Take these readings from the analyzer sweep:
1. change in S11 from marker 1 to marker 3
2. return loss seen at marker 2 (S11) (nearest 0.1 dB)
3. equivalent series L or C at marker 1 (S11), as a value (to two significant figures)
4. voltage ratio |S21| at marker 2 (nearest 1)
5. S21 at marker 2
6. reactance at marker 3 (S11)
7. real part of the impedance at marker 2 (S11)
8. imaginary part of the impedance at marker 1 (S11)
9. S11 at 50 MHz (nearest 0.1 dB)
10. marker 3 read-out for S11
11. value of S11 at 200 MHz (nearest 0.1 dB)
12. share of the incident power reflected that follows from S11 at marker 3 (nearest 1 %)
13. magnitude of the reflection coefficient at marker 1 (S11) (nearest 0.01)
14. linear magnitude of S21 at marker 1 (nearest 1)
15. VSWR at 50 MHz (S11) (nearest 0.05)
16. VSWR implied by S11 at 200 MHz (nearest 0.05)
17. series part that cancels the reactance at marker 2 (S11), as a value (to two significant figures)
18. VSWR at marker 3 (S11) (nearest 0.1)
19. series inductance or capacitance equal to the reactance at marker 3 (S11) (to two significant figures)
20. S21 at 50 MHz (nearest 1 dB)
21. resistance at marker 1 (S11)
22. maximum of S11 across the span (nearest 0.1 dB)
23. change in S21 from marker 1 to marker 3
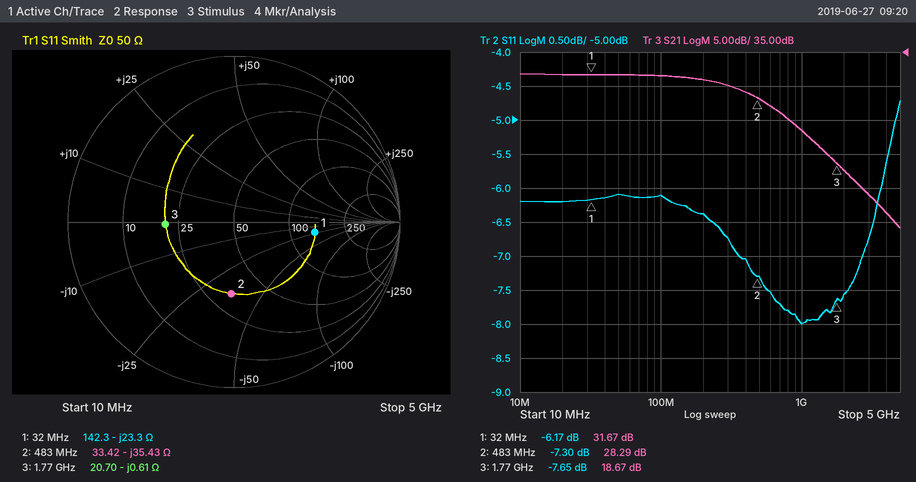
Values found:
-1.48 dB
7.3 dB
210 pF
26
28.29 dB
-0.61 Ω
33.42 Ω
-23.3 Ω
-6.1 dB
-7.65 dB
-6.4 dB
17 %
0.49
38
2.95
2.85
12 nH
2.4
150 pF
32 dB
142.3 Ω
-4.7 dB
-13.00 dB
